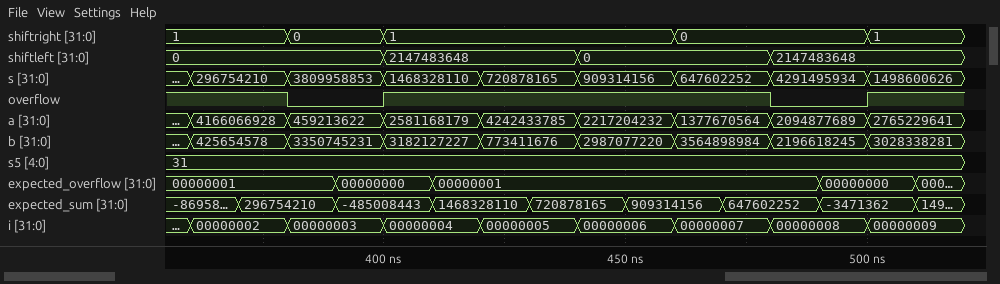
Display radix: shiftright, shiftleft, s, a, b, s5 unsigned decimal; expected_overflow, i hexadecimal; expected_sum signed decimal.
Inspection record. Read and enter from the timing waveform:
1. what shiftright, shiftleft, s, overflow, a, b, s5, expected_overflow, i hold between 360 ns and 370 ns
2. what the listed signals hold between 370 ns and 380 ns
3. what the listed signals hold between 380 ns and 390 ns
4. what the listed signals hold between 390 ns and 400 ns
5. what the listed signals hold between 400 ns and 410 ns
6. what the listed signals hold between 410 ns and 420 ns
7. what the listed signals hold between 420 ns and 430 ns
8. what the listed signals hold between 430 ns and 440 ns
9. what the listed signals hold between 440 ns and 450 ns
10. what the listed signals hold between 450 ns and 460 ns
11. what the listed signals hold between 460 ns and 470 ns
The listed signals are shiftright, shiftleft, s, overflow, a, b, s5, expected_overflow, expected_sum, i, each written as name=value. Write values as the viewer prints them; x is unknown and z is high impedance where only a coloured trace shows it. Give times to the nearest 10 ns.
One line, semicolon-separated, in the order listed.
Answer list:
shiftright=1, shiftleft=0, s=296754210, overflow=1, a=4166066928, b=425654578, s5=31, expected_overflow=00000001, i=00000002; shiftright=1, shiftleft=0, s=296754210, overflow=1, a=4166066928, b=425654578, s5=31, expected_overflow=00000001, expected_sum=296754210, i=00000002; shiftright=0, shiftleft=0, s=3809958853, overflow=0, a=459213622, b=3350745231, s5=31, expected_overflow=00000001, expected_sum=296754210, i=00000003; shiftright=0, shiftleft=0, s=3809958853, overflow=0, a=459213622, b=3350745231, s5=31, expected_overflow=00000000, expected_sum=-485008443, i=00000003; shiftright=1, shiftleft=2147483648, s=1468328110, overflow=1, a=2581168179, b=3182127227, s5=31, expected_overflow=00000000, expected_sum=-485008443, i=00000004; shiftright=1, shiftleft=2147483648, s=1468328110, overflow=1, a=2581168179, b=3182127227, s5=31, expected_overflow=00000001, expected_sum=1468328110, i=00000004; shiftright=1, shiftleft=2147483648, s=720878165, overflow=1, a=4242433785, b=773411676, s5=31, expected_overflow=00000001, expected_sum=1468328110, i=00000005; shiftright=1, shiftleft=2147483648, s=720878165, overflow=1, a=4242433785, b=773411676, s5=31, expected_overflow=00000001, expected_sum=720878165, i=00000005; shiftright=1, shiftleft=0, s=909314156, overflow=1, a=2217204232, b=2987077220, s5=31, expected_overflow=00000001, expected_sum=720878165, i=00000006; shiftright=1, shiftleft=0, s=909314156, overflow=1, a=2217204232, b=2987077220, s5=31, expected_overflow=00000001, expected_sum=909314156, i=00000006; shiftright=0, shiftleft=0, s=647602252, overflow=1, a=1377670564, b=3564898984, s5=31, expected_overflow=00000001, expected_sum=909314156, i=00000007
